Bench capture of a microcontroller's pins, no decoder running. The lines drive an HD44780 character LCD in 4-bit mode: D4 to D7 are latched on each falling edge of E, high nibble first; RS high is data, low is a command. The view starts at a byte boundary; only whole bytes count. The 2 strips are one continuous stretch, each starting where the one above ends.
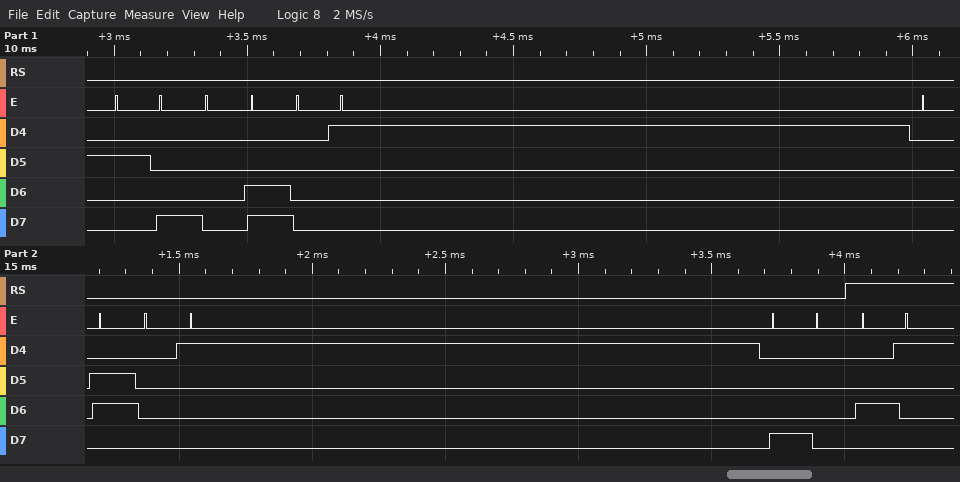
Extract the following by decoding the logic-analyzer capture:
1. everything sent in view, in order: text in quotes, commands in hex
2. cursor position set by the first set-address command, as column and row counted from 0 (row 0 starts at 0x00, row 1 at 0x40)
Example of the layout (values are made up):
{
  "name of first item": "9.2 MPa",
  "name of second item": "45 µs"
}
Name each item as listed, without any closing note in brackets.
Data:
{
  "everything sent in view, in order: text in quotes, commands in hex": "0x28 0x0C 0x01 0x06 0x01 0x80 \"A\"",
  "cursor position set by the first set-address command, as column and row counted from 0": "column 0, row 0"
}
